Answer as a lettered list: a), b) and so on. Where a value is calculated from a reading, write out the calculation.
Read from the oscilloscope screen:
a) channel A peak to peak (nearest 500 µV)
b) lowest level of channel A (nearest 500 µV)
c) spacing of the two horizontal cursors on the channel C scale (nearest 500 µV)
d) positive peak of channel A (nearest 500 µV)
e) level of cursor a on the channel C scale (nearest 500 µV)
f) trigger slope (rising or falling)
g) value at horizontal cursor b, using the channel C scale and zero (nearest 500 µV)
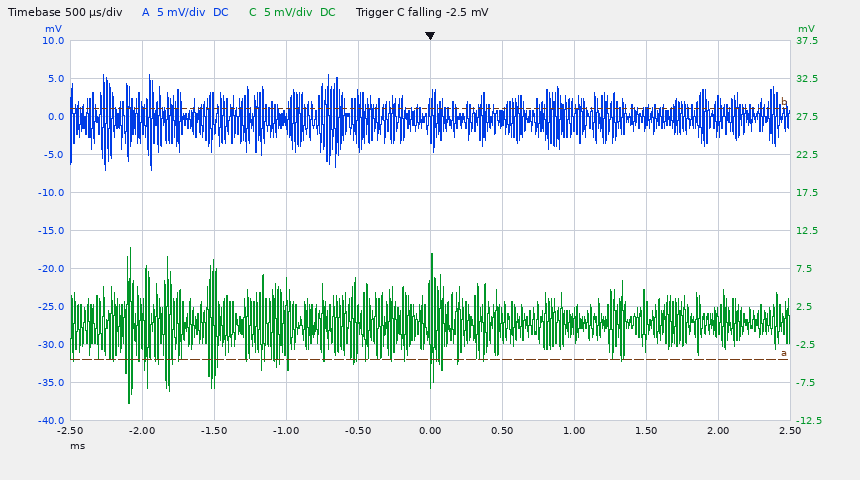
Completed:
a) 5.5 mV − (-7.0 mV) = 12.5 mV
b) -7.0 mV
c) 33.0 mV
d) 5.5 mV
e) -4.5 mV
f) falling
g) 28.5 mV
